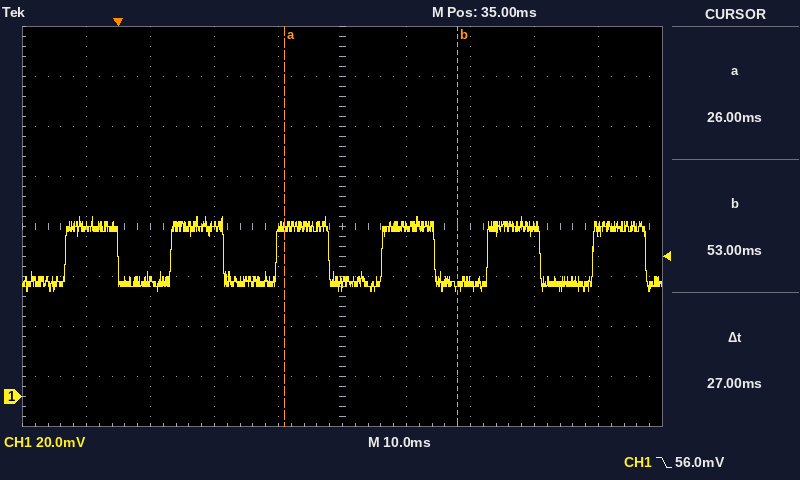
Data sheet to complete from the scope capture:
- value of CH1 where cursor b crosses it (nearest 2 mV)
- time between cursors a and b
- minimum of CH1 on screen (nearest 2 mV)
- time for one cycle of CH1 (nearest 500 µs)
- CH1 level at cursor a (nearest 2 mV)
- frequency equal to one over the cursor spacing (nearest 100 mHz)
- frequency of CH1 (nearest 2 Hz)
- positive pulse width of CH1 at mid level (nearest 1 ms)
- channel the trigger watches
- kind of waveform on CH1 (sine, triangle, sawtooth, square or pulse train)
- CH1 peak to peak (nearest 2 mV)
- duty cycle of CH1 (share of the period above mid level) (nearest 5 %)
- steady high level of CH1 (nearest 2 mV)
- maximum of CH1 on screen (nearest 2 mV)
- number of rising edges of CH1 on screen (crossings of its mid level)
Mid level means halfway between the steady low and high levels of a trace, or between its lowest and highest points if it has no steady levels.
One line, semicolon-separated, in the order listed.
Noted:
44 mV; 27 ms; 42 mV; 16.5 ms; 68 mV; 37.0 Hz; 60 Hz; 8 ms; CH1; square; 30 mV; 50 %; 68 mV; 72 mV; 6
